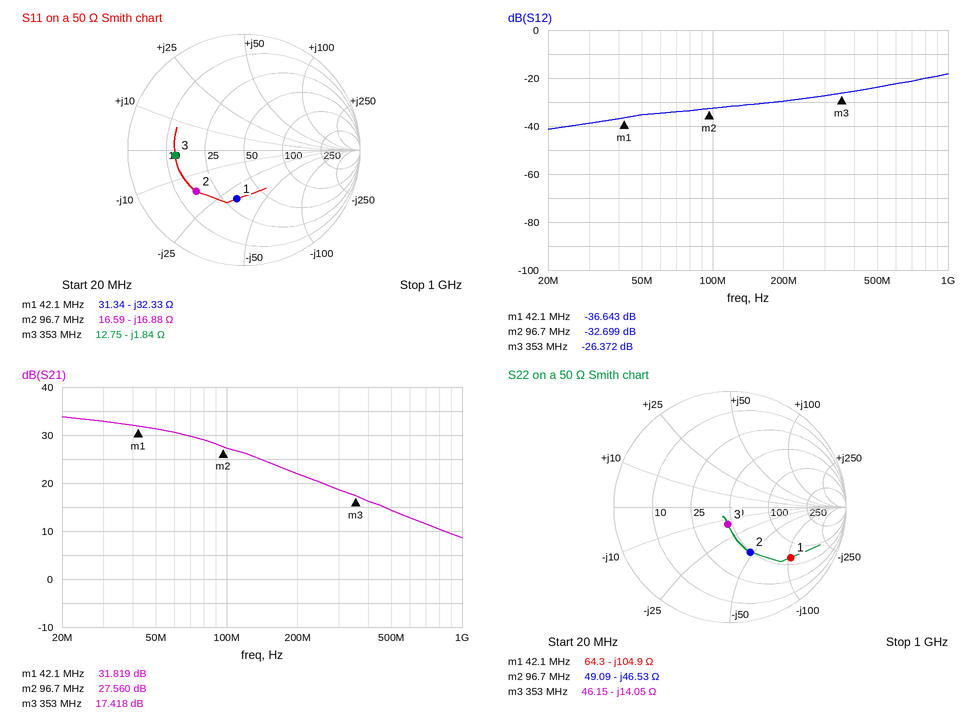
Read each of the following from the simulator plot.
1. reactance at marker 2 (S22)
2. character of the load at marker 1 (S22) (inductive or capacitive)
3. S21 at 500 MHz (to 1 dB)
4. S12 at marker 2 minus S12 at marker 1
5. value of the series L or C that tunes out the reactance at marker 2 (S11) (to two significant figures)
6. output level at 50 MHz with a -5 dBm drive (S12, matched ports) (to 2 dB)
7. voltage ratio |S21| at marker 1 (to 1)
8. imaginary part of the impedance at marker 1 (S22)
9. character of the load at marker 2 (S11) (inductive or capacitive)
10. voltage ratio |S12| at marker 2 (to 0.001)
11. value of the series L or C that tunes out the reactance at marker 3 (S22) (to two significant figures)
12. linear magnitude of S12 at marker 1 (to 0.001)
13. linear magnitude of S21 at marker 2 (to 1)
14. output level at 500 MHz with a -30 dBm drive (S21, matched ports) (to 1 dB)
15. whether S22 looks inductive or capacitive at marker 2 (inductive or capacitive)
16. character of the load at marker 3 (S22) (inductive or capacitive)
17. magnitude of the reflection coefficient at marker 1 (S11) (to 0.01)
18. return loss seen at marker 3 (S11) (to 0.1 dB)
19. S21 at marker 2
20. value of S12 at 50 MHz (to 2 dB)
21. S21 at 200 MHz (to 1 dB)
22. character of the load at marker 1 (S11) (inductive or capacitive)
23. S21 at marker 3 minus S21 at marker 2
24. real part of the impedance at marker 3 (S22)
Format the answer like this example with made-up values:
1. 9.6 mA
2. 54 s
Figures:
1. -46.53 Ω
2. capacitive
3. 14 dB
4. 3.944 dB
5. 28 nH
6. -40 dBm
7. 39
8. -104.9 Ω
9. capacitive
10. 0.023
11. 6.3 nH
12. 0.015
13. 24
14. -16 dBm
15. capacitive
16. capacitive
17. 0.43
18. 4.5 dB
19. 27.560 dB
20. -36 dB
21. 22 dB
22. capacitive
23. -10.142 dB
24. 46.15 Ω
